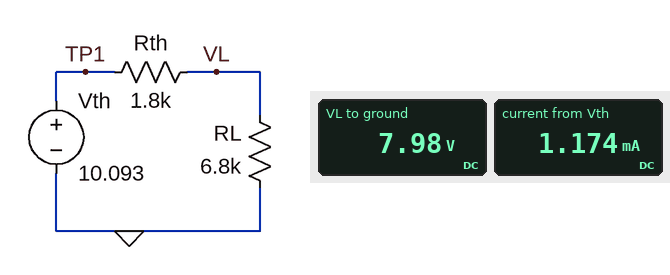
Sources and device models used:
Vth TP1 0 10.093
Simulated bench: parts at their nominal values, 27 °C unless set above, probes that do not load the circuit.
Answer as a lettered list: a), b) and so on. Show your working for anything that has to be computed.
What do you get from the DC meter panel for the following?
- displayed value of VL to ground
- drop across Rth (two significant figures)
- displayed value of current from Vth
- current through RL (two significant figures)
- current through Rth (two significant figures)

a) 7.98 V
b) 10.09 V - 7.98 V = 2.1 V
c) 1.174 mA
d) (7.98 V) / 6.8 kΩ = 1.2 mA
e) (10.09 V - 7.98 V) / 1.8 kΩ = 1.2 mA
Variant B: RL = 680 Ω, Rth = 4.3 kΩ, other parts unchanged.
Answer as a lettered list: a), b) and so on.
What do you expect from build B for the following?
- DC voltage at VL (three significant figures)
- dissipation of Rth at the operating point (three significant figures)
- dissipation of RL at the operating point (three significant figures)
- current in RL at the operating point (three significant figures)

a) 1.38 V
b) 17.7 mW
c) 2.79 mW
d) 2.03 mA
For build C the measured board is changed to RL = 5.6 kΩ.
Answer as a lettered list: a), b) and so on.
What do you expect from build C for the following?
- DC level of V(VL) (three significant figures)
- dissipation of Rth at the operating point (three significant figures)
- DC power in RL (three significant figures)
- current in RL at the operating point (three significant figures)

a) 7.64 V
b) 3.35 mW
c) 10.4 mW
d) 1.36 mA
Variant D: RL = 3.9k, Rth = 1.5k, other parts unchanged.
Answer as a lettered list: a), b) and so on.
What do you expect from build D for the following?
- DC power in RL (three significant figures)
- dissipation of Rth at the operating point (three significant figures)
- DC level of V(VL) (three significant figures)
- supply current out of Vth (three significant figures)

a) 13.6 mW
b) 5.24 mW
c) 7.29 V
d) 1.87 mA
